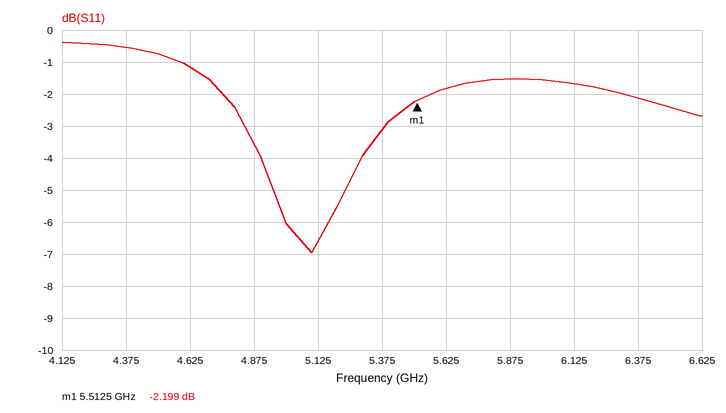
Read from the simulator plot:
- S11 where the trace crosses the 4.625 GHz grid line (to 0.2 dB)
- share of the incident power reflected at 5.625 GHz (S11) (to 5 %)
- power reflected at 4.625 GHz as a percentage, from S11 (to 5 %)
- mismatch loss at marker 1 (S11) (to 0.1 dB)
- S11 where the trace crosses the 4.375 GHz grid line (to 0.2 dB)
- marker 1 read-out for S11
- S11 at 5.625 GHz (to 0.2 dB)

-1.2 dB
65 %
75 %
4.0 dB
-0.6 dB
-2.199 dB
-1.8 dB
